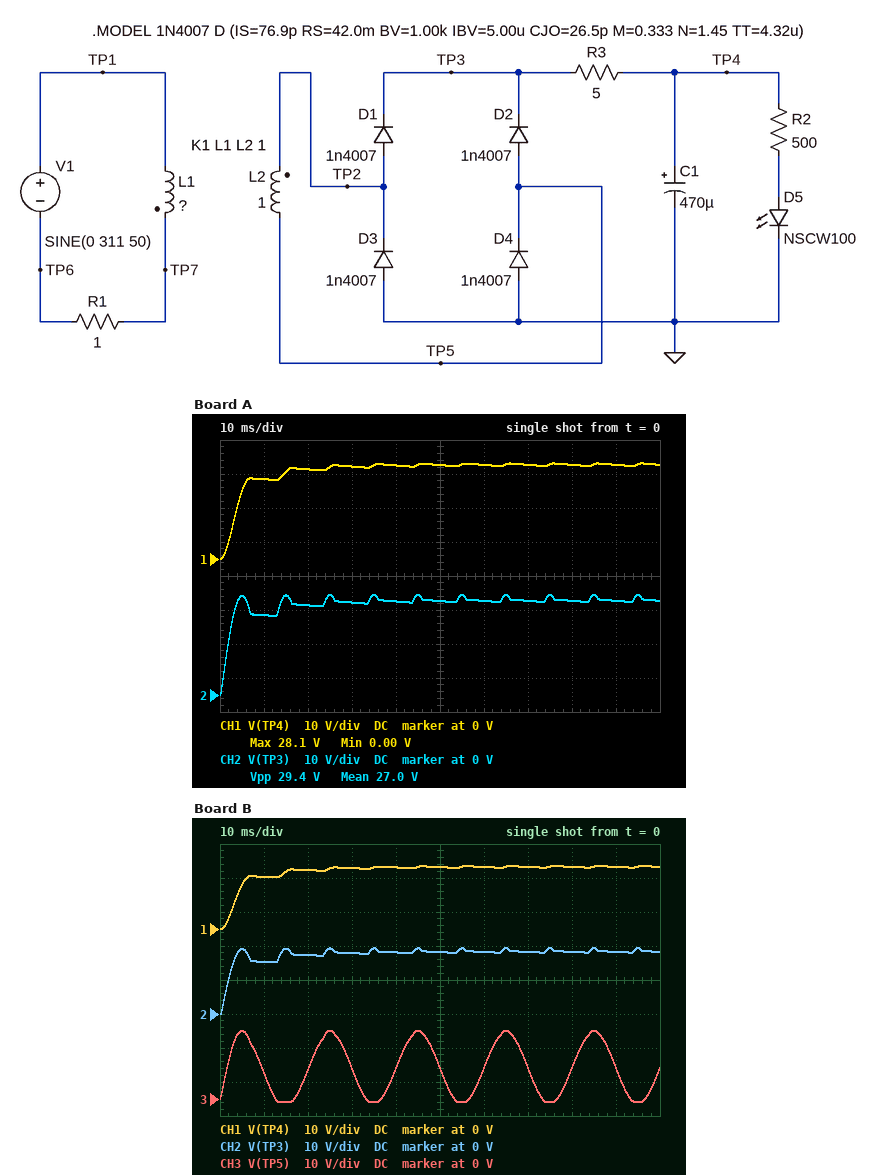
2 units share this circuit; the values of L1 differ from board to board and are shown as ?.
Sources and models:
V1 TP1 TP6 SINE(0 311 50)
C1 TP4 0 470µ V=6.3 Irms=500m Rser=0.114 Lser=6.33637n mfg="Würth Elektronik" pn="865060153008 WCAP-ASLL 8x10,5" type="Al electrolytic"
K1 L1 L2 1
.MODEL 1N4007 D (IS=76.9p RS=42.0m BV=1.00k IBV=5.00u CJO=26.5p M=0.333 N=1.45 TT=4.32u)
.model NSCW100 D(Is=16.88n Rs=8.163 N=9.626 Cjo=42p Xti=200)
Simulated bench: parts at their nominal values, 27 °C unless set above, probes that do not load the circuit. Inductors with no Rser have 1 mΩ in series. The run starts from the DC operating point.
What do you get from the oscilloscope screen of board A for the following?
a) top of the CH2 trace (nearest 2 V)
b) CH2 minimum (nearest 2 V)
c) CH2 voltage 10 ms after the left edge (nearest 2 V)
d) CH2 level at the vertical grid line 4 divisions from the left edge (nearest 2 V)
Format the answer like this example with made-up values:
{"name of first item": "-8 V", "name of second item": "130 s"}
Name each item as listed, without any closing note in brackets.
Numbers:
{"top of the CH2 trace": "30 V", "CH2 minimum": "0 V", "CH2 voltage 10 ms after the left edge": "24 V", "CH2 level at the vertical grid line 4 divisions from the left edge": "28 V"}
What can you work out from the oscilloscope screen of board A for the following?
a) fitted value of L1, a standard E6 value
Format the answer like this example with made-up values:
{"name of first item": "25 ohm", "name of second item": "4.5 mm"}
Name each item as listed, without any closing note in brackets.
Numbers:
{"fitted value of L1, a standard E6 value": "100 H"}
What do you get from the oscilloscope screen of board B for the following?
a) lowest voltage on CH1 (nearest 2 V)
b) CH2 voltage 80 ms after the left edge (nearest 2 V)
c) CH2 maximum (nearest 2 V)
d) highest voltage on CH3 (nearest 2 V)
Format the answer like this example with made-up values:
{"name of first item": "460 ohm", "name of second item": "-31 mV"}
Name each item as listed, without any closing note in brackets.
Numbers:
{"lowest voltage on CH1": "0 V", "CH2 voltage 80 ms after the left edge": "18 V", "CH2 maximum": "20 V", "highest voltage on CH3": "20 V"}
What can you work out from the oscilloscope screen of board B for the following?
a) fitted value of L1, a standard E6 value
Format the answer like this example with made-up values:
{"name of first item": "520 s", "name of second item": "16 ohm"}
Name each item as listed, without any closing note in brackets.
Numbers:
{"fitted value of L1, a standard E6 value": "220 H"}
